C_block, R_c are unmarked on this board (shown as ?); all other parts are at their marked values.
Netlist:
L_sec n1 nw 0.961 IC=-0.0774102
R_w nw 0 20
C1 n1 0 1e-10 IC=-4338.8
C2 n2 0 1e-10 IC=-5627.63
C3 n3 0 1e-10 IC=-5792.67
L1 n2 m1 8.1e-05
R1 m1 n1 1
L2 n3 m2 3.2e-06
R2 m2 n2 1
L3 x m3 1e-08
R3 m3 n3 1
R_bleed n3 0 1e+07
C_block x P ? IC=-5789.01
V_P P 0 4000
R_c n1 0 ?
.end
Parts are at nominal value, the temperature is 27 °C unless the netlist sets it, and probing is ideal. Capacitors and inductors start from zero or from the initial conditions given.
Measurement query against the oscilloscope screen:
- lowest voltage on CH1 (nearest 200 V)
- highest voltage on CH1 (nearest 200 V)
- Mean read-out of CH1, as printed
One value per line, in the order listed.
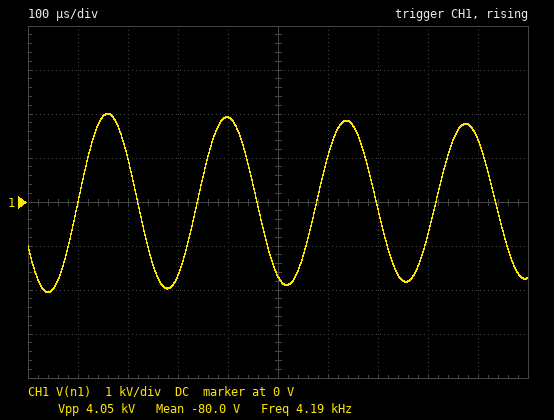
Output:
-2.0 kV
2.0 kV
-80.0 V
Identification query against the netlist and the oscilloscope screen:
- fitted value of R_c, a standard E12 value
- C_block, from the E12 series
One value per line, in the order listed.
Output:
2.7 MΩ
1.2 nF
